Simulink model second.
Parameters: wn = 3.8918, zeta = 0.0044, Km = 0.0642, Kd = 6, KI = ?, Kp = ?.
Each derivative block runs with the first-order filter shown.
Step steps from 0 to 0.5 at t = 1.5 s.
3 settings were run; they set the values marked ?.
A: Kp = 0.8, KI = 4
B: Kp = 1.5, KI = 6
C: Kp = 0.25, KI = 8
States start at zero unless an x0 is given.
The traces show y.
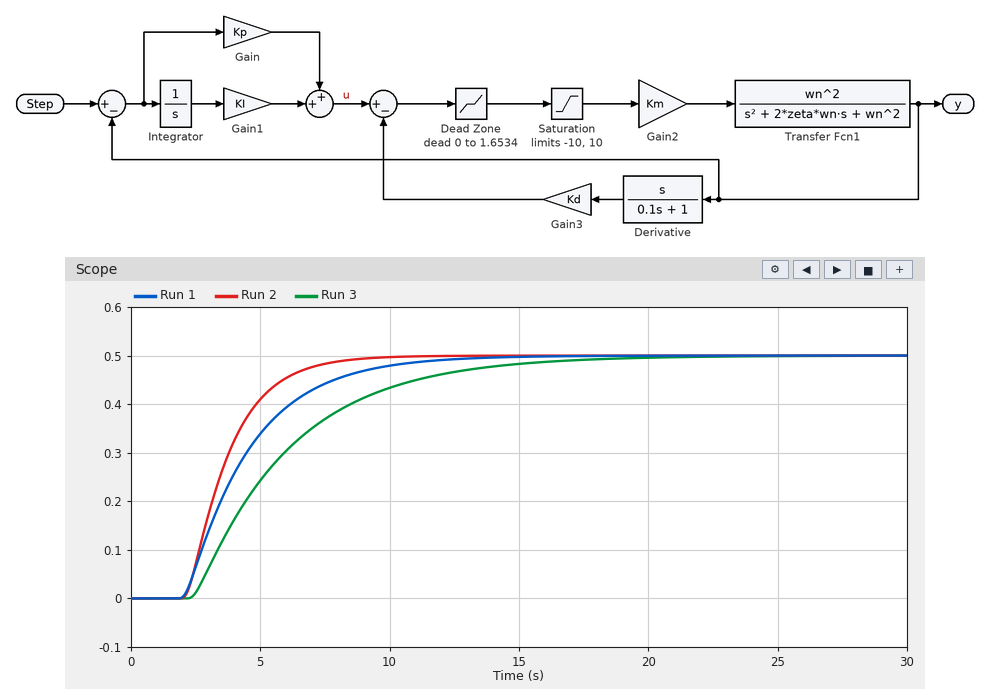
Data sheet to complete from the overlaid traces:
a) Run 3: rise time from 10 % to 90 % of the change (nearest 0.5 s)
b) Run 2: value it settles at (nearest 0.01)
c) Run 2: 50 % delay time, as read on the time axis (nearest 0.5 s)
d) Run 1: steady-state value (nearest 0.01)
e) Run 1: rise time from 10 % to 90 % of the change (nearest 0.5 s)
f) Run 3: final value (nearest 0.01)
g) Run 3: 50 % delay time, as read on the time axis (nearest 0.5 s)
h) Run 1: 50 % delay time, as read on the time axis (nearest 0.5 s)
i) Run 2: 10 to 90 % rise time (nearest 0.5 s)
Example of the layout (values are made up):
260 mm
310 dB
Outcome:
8.0 s
0.50
3.5 s
0.50
5.5 s
0.50
5.0 s
4.0 s
3.5 s
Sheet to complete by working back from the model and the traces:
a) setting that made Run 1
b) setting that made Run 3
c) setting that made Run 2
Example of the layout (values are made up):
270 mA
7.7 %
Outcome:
B
A
C
